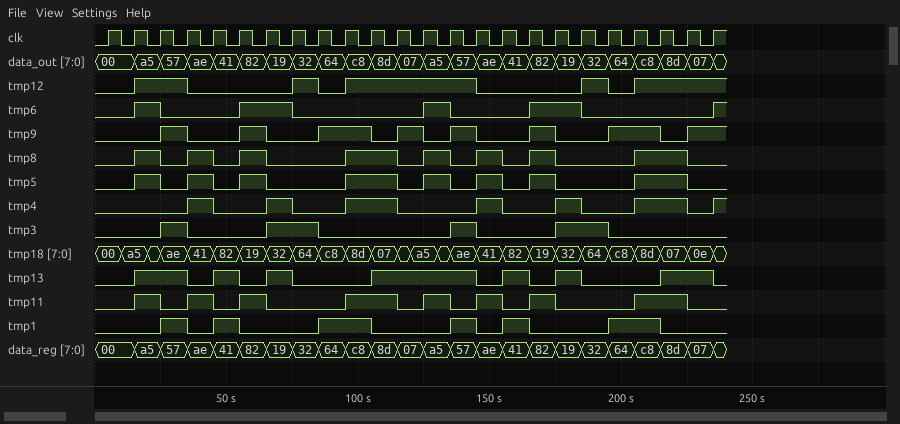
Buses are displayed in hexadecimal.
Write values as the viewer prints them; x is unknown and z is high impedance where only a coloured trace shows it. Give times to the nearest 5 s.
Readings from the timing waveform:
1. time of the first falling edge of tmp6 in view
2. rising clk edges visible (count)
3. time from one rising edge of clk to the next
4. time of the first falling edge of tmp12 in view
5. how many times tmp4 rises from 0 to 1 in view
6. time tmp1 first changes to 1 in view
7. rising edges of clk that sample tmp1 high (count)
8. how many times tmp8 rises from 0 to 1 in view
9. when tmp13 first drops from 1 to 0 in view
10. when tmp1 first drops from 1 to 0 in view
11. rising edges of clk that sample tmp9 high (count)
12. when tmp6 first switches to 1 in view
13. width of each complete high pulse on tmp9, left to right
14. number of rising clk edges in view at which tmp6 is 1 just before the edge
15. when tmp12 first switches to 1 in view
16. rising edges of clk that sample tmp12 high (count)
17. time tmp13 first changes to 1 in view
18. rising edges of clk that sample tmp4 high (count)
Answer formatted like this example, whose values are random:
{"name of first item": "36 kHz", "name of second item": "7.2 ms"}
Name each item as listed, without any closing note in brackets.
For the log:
{"time of the first falling edge of tmp6 in view": "25 s", "rising clk edges visible": "24", "time from one rising edge of clk to the next": "10 s", "time of the first falling edge of tmp12 in view": "35 s", "how many times tmp4 rises from 0 to 1 in view": "7", "time tmp1 first changes to 1 in view": "25 s", "rising edges of clk that sample tmp1 high": "8", "how many times tmp8 rises from 0 to 1 in view": "8", "when tmp13 first drops from 1 to 0 in view": "35 s", "when tmp1 first drops from 1 to 0 in view": "35 s", "rising edges of clk that sample tmp9 high": "10", "when tmp6 first switches to 1 in view": "15 s", "width of each complete high pulse on tmp9, left to right": "10 s, 10 s, 20 s, 10 s, 10 s, 10 s, 20 s", "number of rising clk edges in view at which tmp6 is 1 just before the edge": "6", "when tmp12 first switches to 1 in view": "15 s", "rising edges of clk that sample tmp12 high": "12", "time tmp13 first changes to 1 in view": "15 s", "rising edges of clk that sample tmp4 high": "8"}
